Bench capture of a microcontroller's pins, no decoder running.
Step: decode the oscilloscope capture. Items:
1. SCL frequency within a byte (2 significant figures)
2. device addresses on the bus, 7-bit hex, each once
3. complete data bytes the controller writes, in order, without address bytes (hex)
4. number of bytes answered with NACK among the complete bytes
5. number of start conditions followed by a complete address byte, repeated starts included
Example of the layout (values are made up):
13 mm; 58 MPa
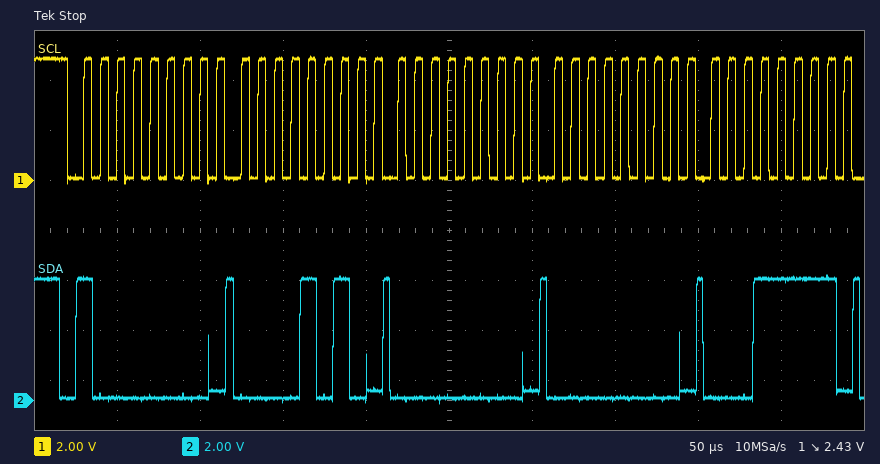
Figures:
100 kHz; 0x40; 0A 00 00 1F; 0; 1
